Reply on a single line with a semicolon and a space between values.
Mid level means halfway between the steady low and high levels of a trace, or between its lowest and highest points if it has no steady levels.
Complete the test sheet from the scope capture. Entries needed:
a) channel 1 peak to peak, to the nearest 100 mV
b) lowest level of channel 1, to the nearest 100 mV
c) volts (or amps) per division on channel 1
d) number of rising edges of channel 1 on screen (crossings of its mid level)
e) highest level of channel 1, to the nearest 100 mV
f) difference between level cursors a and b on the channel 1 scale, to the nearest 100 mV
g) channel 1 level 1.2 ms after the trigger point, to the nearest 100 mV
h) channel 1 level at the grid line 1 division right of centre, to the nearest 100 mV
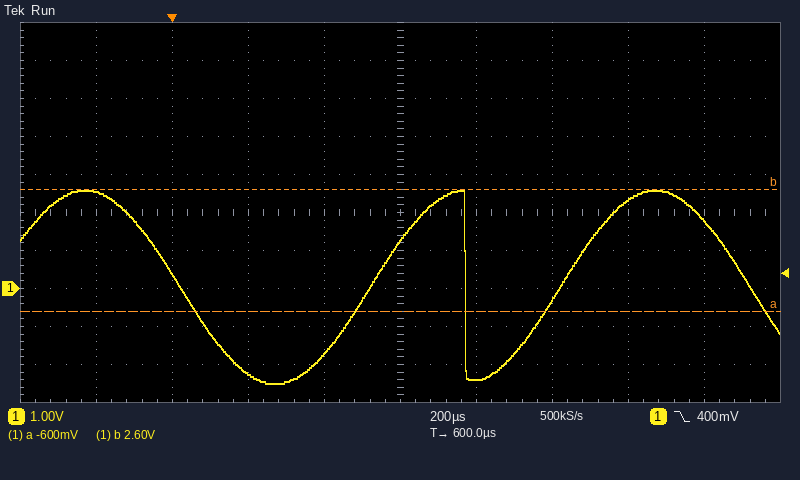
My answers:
5.1 V; -2.5 V; 1 V; 2; 2.6 V; 3.2 V; 2.3 V; -2.4 V
